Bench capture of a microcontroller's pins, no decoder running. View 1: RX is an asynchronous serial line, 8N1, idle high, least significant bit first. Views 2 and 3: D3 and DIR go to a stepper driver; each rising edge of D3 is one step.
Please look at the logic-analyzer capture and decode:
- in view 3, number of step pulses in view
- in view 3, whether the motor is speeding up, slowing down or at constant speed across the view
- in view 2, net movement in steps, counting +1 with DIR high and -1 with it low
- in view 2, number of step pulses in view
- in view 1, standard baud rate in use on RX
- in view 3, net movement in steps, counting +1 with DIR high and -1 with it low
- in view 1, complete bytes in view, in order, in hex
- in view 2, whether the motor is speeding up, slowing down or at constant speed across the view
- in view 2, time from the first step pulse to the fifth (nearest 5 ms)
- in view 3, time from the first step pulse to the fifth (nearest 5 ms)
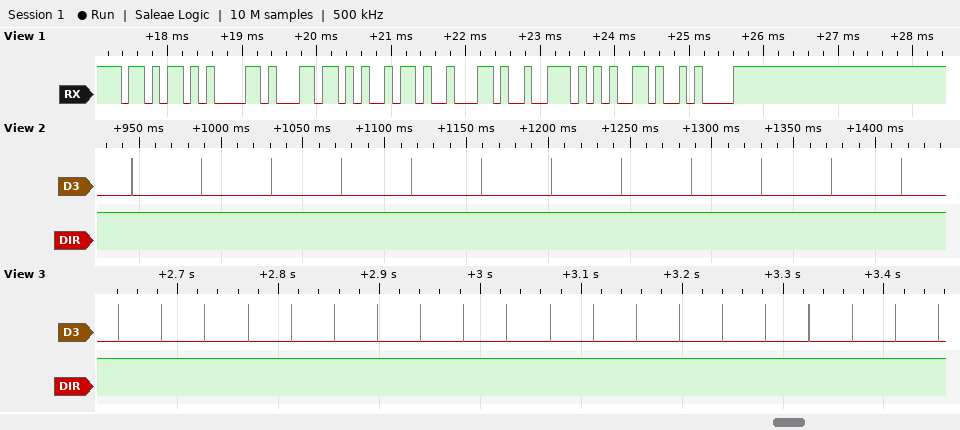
20
constant speed
+12
12
9600 baud
+20
0x6B 0x61 0x6C 0x69 0x62 0x72 0x65 0x0A
constant speed
170 ms
170 ms
